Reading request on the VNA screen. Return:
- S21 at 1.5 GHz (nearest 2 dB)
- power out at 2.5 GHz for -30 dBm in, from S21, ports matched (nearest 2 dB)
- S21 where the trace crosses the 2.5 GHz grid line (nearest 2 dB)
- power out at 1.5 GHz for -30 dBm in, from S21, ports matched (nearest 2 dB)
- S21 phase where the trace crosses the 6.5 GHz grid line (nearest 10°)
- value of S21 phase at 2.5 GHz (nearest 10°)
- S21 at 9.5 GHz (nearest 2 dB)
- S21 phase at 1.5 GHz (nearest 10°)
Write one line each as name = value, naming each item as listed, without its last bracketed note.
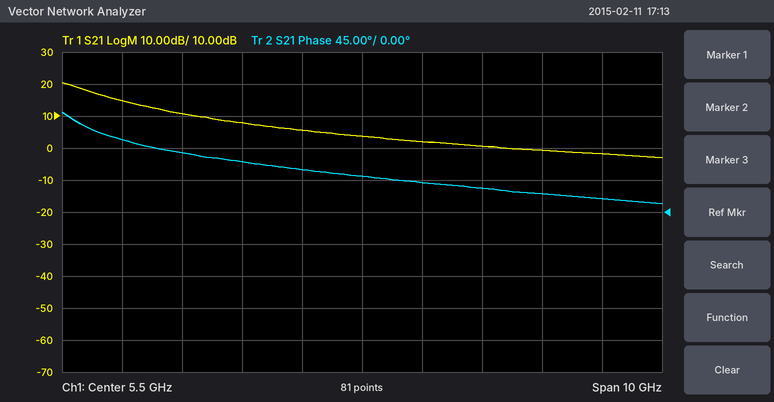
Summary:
S21 at 1.5 GHz = 14 dB
power out at 2.5 GHz for -30 dBm in, from S21, ports matched = -20 dBm
S21 where the trace crosses the 2.5 GHz grid line = 10 dB
power out at 1.5 GHz for -30 dBm in, from S21, ports matched = -16 dBm
S21 phase where the trace crosses the 6.5 GHz grid line = 40°
value of S21 phase at 2.5 GHz = 80°
S21 at 9.5 GHz = -2 dB
S21 phase at 1.5 GHz = 100°
